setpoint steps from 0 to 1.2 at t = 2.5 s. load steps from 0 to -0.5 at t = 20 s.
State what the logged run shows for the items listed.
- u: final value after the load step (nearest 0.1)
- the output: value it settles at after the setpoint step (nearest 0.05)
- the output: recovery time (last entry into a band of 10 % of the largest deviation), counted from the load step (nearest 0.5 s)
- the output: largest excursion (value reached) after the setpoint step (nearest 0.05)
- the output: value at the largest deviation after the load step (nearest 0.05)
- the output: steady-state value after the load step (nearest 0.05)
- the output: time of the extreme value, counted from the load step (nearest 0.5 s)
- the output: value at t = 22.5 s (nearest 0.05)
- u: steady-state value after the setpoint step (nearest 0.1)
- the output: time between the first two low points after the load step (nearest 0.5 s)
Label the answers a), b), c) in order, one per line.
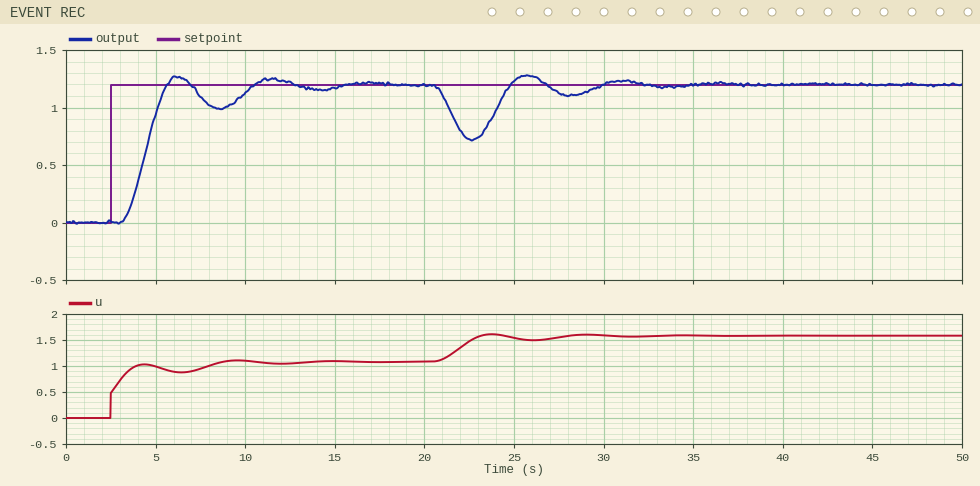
a) 1.6
b) 1.20
c) 9.5 s
d) 1.25
e) 0.70
f) 1.20
g) 2.5 s
h) 0.70
i) 1.1
j) 5.5 s
